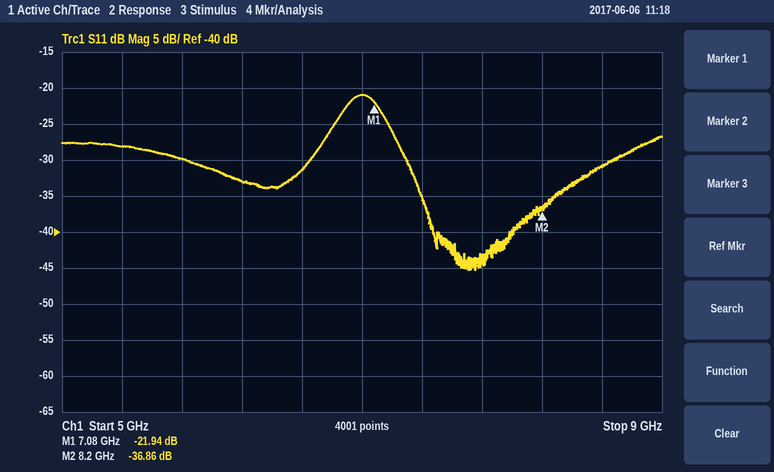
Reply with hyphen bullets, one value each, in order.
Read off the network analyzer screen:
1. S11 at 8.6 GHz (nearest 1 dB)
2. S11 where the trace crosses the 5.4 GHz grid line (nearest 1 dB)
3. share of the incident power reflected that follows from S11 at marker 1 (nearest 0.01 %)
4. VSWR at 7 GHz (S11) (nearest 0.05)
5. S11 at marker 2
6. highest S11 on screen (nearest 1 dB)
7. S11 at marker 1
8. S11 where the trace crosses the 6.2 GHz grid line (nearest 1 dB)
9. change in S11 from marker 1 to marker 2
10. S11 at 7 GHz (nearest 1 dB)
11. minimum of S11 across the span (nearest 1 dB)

- -31 dB
- -28 dB
- 0.64 %
- 1.20
- -36.86 dB
- -21 dB
- -21.94 dB
- -33 dB
- -14.92 dB
- -21 dB
- -45 dB
